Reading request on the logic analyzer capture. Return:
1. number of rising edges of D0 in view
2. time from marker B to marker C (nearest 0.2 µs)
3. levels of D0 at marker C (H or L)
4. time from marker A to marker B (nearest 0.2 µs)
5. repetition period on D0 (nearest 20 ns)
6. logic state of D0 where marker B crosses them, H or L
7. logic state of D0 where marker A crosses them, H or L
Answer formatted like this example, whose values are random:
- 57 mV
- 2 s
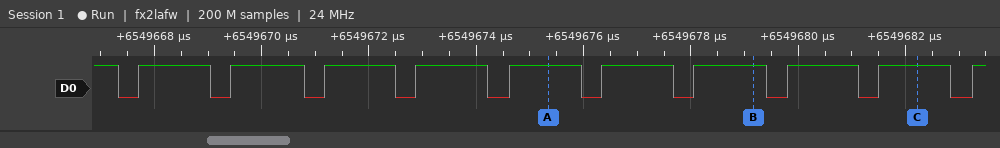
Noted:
- 10
- 3 µs
- D0=H
- 3.8 µs
- 1720 ns
- D0=H
- D0=H
